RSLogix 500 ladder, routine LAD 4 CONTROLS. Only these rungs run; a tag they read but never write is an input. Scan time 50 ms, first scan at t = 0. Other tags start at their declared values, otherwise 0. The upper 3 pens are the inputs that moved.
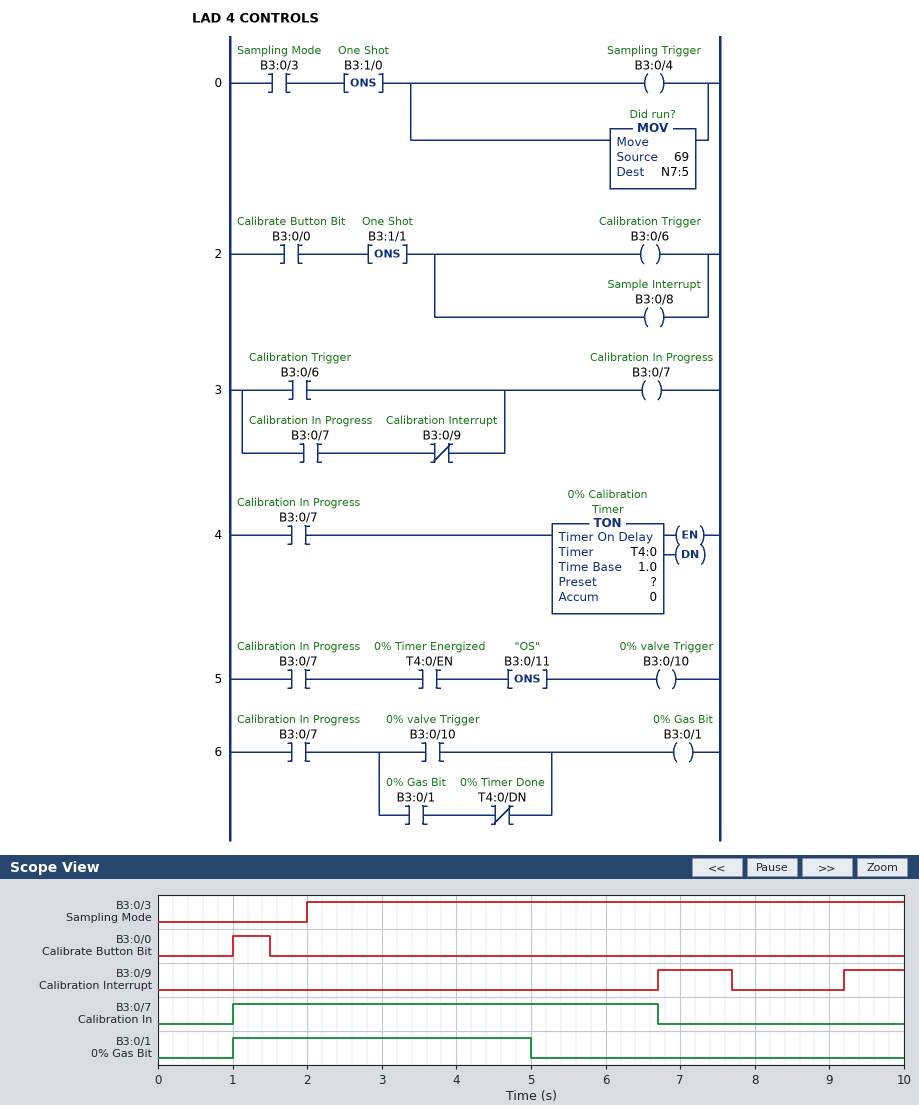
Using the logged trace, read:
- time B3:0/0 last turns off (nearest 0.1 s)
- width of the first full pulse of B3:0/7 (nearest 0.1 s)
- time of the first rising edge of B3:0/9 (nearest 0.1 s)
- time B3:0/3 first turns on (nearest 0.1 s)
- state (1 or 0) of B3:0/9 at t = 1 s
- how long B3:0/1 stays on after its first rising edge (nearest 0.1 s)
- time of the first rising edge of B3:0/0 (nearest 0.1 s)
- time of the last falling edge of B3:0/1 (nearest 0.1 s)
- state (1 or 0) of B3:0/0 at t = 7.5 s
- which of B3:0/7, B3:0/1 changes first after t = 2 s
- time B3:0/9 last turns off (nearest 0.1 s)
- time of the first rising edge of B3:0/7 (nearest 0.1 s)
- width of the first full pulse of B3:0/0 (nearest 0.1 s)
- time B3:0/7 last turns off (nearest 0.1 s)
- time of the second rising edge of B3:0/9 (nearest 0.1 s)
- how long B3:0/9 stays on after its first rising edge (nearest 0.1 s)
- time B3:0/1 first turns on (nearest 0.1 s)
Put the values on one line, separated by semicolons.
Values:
1.5 s; 5.7 s; 6.7 s; 2.0 s; 0; 4.0 s; 1.0 s; 5.0 s; 0; B3:0/1; 7.7 s; 1.0 s; 0.5 s; 6.7 s; 9.2 s; 1.0 s; 1.0 s
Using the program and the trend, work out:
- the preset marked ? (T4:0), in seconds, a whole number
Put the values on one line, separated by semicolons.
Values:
4 s
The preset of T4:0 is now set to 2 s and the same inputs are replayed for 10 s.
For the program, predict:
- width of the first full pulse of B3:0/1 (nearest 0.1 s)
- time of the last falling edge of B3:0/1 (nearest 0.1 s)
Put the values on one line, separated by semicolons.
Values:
2.0 s; 3.0 s
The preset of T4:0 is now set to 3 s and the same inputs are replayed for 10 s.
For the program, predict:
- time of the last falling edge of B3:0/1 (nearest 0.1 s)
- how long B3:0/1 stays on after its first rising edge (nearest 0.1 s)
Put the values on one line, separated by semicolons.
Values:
4.0 s; 3.0 s
